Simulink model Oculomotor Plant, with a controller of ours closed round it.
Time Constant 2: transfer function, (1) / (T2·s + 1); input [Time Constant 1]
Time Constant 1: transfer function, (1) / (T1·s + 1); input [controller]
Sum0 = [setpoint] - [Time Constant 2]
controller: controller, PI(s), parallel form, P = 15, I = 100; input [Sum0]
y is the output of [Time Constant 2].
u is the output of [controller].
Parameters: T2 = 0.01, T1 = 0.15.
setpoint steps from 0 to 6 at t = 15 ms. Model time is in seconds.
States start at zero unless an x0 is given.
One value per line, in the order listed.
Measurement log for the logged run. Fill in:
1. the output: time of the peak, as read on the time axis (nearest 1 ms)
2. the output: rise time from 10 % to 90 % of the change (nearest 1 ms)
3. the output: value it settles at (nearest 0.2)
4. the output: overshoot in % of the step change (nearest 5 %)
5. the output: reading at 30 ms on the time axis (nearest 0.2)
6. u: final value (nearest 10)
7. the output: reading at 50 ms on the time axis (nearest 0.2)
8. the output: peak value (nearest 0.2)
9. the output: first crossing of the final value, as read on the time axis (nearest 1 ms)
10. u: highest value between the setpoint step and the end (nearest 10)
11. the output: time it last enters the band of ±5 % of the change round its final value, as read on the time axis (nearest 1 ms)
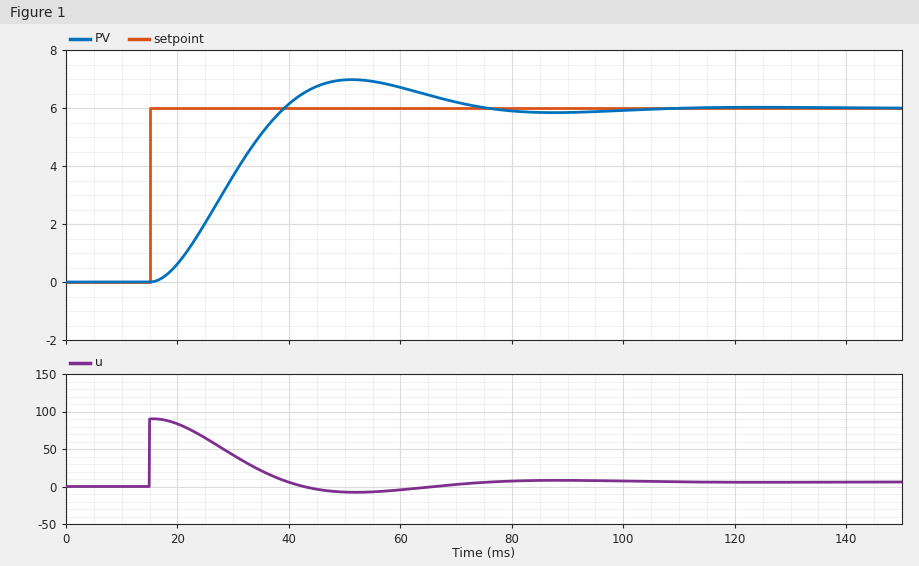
51 ms
16 ms
6.0
15 %
3.6
10
7.0
7.0
39 ms
90
68 ms
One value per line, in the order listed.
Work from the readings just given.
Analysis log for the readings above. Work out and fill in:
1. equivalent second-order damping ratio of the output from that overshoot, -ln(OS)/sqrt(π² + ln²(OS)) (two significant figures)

0.52
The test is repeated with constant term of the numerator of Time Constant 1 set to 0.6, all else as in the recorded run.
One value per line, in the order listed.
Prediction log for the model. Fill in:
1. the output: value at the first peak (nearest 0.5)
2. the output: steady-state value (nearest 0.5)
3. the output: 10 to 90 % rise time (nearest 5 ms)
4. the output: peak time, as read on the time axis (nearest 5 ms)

6.5
6.0
25 ms
70 ms
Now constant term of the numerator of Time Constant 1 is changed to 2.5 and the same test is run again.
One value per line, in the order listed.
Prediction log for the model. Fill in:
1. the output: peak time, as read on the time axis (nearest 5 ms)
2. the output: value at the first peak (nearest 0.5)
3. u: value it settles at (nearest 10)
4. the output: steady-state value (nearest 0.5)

35 ms
8.0
0
6.0
